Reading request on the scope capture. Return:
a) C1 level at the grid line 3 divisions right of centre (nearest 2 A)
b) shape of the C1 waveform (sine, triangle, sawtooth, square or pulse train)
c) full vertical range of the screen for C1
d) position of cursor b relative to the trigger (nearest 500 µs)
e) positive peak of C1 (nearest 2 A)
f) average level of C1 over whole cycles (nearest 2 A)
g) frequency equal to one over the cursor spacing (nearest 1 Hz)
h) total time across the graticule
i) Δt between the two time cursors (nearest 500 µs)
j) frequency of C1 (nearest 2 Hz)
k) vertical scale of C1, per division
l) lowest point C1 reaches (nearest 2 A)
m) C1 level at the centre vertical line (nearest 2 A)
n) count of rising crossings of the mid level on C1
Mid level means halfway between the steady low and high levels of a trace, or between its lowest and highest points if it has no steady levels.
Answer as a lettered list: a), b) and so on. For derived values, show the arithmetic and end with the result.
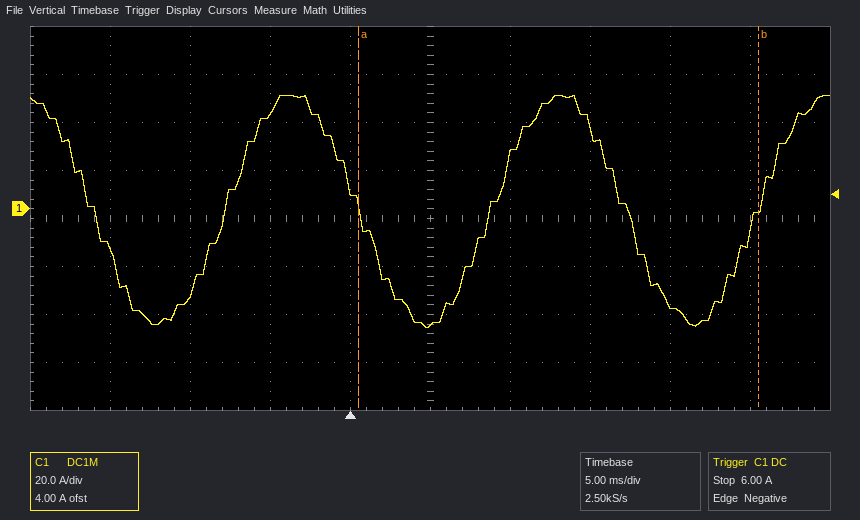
a) -40 A
b) sine
c) 160 A
d) +25.5 ms
e) 48 A
f) (48 A + (-50 A)) / 2 ≈ 0 A
g) 1 / 25.0 ms ≈ 40 Hz
h) 50 ms
i) 25.0 ms
j) 60 Hz
k) 20 A
l) -50 A
m) -48 A
n) 3
